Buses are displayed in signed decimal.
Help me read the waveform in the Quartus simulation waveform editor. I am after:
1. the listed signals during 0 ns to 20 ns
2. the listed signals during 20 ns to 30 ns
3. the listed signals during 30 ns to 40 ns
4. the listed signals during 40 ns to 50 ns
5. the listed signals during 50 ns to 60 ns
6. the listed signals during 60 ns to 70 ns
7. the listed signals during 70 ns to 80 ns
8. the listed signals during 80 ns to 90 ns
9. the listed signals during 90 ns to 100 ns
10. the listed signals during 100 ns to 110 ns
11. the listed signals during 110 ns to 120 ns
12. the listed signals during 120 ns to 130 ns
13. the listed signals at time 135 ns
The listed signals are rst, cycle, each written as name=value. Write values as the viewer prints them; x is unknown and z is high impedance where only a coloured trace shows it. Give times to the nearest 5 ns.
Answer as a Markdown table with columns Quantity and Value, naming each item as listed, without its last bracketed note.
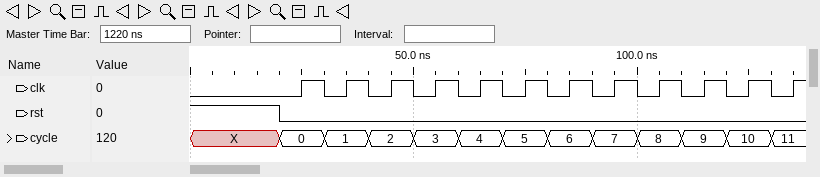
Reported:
| Quantity | Value |
|---|---|
| the listed signals during 0 ns to 20 ns | rst=1, cycle=X |
| the listed signals during 20 ns to 30 ns | rst=0, cycle=0 |
| the listed signals during 30 ns to 40 ns | rst=0, cycle=1 |
| the listed signals during 40 ns to 50 ns | rst=0, cycle=2 |
| the listed signals during 50 ns to 60 ns | rst=0, cycle=3 |
| the listed signals during 60 ns to 70 ns | rst=0, cycle=4 |
| the listed signals during 70 ns to 80 ns | rst=0, cycle=5 |
| the listed signals during 80 ns to 90 ns | rst=0, cycle=6 |
| the listed signals during 90 ns to 100 ns | rst=0, cycle=7 |
| the listed signals during 100 ns to 110 ns | rst=0, cycle=8 |
| the listed signals during 110 ns to 120 ns | rst=0, cycle=9 |
| the listed signals during 120 ns to 130 ns | rst=0, cycle=10 |
| the listed signals at time 135 ns | rst=0, cycle=11 |
